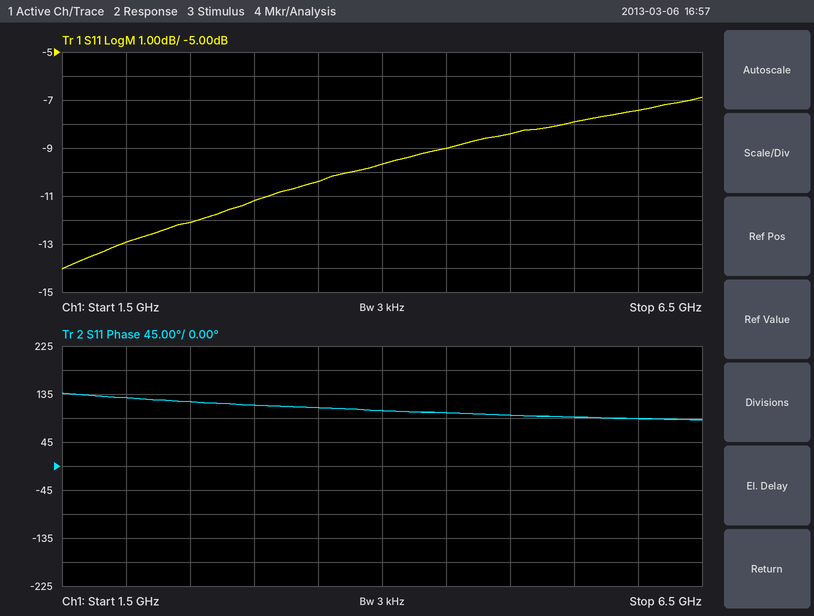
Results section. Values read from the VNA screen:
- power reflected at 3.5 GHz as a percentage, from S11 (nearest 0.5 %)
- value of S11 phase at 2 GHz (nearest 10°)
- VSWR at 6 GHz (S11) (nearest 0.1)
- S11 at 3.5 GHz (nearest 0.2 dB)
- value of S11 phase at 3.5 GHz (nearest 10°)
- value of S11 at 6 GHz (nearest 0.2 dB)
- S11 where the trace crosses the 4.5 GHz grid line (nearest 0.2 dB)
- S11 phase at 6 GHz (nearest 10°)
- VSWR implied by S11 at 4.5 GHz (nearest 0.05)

9.0 %
130°
2.5
-10.4 dB
110°
-7.4 dB
-9.0 dB
90°
2.10
